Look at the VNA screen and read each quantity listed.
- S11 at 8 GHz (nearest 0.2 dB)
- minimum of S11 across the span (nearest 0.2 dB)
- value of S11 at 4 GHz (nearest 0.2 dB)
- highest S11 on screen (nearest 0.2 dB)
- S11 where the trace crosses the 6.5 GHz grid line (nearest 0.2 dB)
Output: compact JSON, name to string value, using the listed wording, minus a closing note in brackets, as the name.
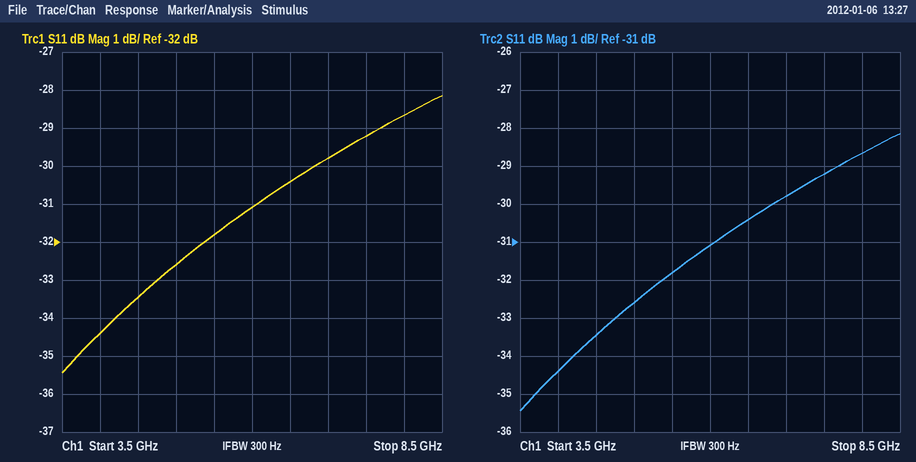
{"S11 at 8 GHz": "-28.6 dB", "minimum of S11 across the span": "-35.4 dB", "value of S11 at 4 GHz": "-34.4 dB", "highest S11 on screen": "-28.2 dB", "S11 where the trace crosses the 6.5 GHz grid line": "-30.4 dB"}
